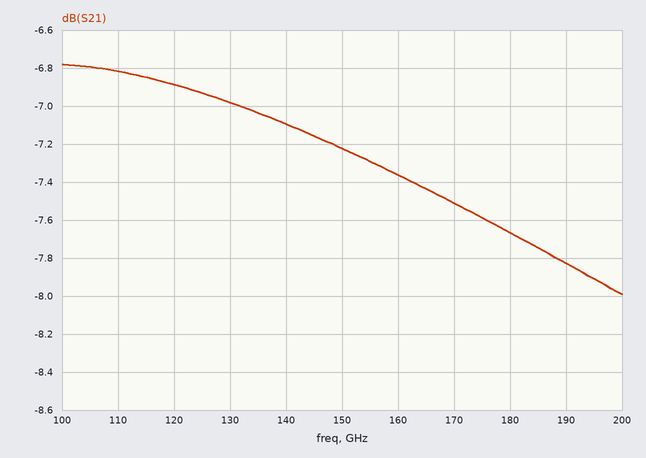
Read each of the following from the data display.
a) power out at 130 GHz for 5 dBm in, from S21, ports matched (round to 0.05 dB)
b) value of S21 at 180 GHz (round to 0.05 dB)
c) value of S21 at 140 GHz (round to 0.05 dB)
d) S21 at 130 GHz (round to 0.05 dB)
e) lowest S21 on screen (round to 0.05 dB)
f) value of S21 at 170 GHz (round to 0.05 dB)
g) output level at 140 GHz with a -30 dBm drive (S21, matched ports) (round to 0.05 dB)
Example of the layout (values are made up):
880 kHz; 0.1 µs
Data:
-2.00 dBm; -7.65 dB; -7.10 dB; -7.00 dB; -8.00 dB; -7.50 dB; -37.10 dBm
